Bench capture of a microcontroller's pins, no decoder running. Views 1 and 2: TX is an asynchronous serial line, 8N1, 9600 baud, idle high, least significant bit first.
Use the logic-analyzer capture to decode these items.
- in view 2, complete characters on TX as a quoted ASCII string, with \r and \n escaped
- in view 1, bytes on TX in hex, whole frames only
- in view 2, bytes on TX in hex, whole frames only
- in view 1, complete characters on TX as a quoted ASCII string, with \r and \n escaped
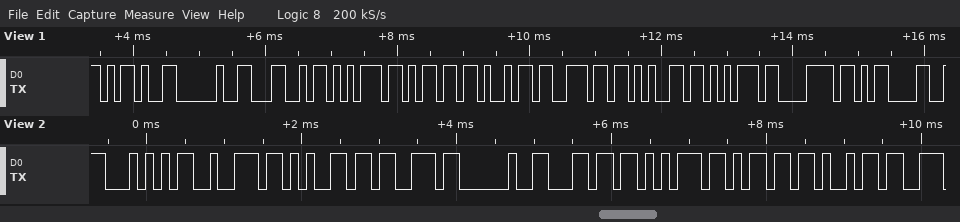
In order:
"Tres lumi"
2D 20 4C 75 6D 69 6E 65 75 78 0D
54 72 65 73 20 6C 75 6D 69
"- Lumineux\r"
